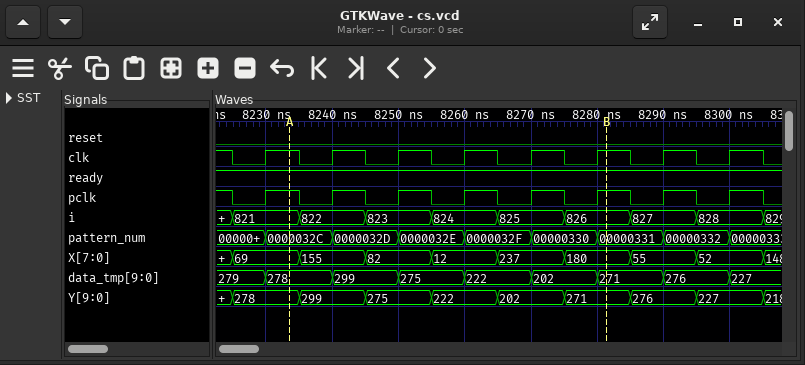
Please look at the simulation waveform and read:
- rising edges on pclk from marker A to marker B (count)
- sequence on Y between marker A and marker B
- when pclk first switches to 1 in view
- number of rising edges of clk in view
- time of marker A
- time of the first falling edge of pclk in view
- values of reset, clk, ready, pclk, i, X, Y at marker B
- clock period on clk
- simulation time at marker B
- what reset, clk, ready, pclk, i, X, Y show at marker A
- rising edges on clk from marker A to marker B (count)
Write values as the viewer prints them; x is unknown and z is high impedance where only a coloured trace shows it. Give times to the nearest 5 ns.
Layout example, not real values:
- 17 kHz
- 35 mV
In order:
- 5
- 278, 299, 275, 222, 202, 271
- 8230 ns
- 8
- 8235 ns
- 8225 ns
- reset=0, clk=1, ready=1, pclk=1, i=826, X=180, Y=271
- 10 ns
- 8280 ns
- reset=0, clk=1, ready=1, pclk=1, i=821, X=69, Y=278
- 5
